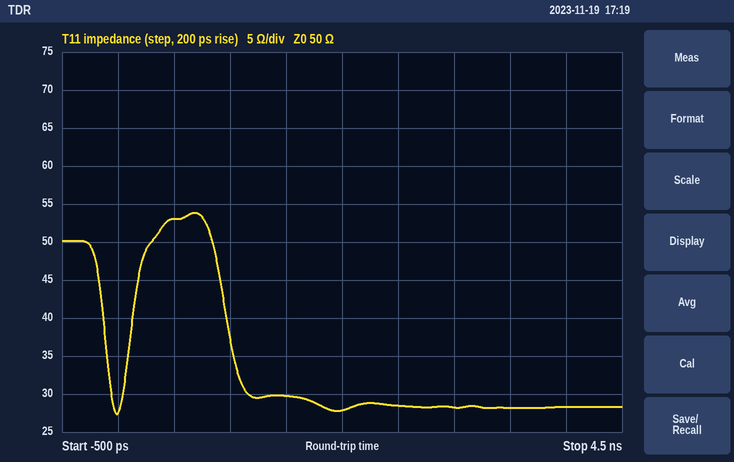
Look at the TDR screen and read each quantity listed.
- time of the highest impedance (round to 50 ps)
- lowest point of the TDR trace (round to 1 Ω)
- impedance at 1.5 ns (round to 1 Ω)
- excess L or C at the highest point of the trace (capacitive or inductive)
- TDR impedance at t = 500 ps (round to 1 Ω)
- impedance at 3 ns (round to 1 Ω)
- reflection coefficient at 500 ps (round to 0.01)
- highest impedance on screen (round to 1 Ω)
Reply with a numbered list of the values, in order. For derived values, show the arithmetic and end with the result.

1. 700 ps
2. 27 Ω
3. 30 Ω
4. inductive
5. 53 Ω
6. 28 Ω
7. (53 − 50)/(53 + 50) ≈ +0.03
8. 54 Ω
